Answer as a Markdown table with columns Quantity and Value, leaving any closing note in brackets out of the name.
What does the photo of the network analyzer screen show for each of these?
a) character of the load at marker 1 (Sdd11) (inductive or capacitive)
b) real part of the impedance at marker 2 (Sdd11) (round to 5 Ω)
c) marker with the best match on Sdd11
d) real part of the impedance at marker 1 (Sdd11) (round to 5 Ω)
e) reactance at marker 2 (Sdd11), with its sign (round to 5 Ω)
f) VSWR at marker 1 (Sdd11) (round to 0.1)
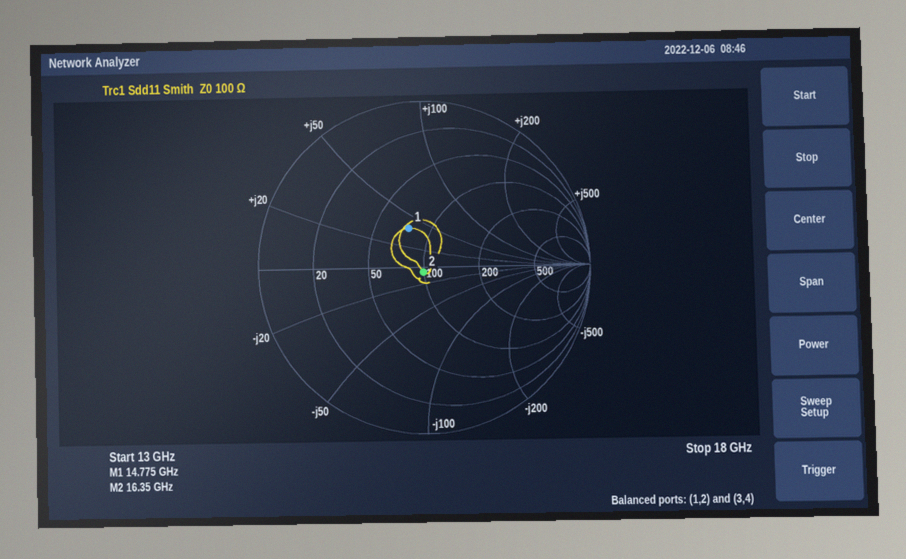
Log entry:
| Quantity | Value |
|---|---|
| character of the load at marker 1 (Sdd11) | inductive |
| real part of the impedance at marker 2 (Sdd11) | 100 Ω |
| marker with the best match on Sdd11 | marker 2 |
| real part of the impedance at marker 1 (Sdd11) | 75 Ω |
| reactance at marker 2 (Sdd11), with its sign | -5 Ω |
| VSWR at marker 1 (Sdd11) | 1.7 |
